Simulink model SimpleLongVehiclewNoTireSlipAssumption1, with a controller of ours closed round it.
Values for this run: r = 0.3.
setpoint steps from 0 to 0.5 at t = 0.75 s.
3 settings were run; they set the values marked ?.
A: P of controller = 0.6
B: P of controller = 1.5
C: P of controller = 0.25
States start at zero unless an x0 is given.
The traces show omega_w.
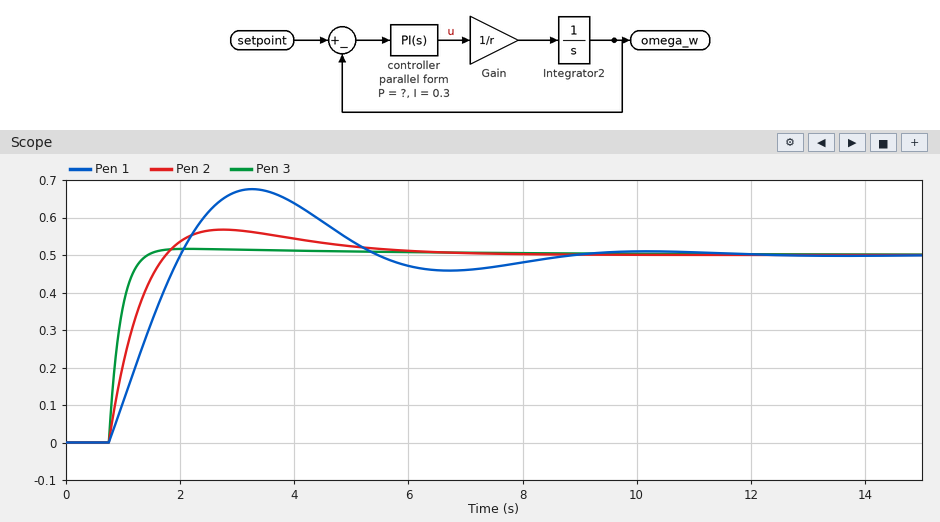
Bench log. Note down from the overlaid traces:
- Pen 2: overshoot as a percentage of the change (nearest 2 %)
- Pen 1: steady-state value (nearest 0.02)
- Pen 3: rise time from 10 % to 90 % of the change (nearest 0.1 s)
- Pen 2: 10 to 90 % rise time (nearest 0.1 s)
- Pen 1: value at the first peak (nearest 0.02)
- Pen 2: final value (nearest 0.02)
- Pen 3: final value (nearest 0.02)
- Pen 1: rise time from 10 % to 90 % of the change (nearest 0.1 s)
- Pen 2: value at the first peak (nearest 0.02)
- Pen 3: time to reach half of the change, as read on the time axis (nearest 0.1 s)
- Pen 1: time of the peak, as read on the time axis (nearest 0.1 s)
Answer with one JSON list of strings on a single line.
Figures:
["14 %", "0.50", "0.4 s", "0.7 s", "0.68", "0.50", "0.50", "1.0 s", "0.56", "0.9 s", "3.3 s"]
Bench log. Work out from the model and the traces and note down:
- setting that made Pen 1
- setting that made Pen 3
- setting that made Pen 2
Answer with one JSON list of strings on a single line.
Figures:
["C", "B", "A"]
